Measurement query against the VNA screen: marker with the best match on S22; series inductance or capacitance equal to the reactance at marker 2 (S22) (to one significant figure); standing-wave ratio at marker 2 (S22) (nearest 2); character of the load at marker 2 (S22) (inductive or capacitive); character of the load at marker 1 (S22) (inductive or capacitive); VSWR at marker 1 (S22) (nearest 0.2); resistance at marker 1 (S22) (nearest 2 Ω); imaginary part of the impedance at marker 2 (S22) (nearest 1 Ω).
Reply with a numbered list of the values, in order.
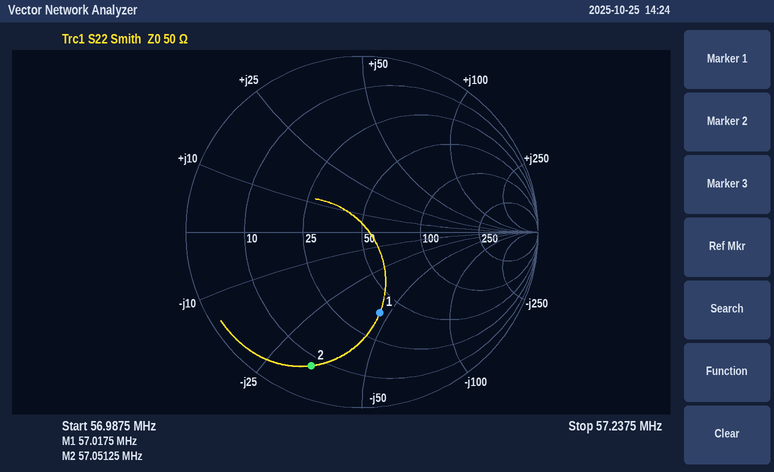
1. marker 1
2. 80 pF
3. 10
4. capacitive
5. capacitive
6. 2.8
7. 38 Ω
8. -34 Ω
